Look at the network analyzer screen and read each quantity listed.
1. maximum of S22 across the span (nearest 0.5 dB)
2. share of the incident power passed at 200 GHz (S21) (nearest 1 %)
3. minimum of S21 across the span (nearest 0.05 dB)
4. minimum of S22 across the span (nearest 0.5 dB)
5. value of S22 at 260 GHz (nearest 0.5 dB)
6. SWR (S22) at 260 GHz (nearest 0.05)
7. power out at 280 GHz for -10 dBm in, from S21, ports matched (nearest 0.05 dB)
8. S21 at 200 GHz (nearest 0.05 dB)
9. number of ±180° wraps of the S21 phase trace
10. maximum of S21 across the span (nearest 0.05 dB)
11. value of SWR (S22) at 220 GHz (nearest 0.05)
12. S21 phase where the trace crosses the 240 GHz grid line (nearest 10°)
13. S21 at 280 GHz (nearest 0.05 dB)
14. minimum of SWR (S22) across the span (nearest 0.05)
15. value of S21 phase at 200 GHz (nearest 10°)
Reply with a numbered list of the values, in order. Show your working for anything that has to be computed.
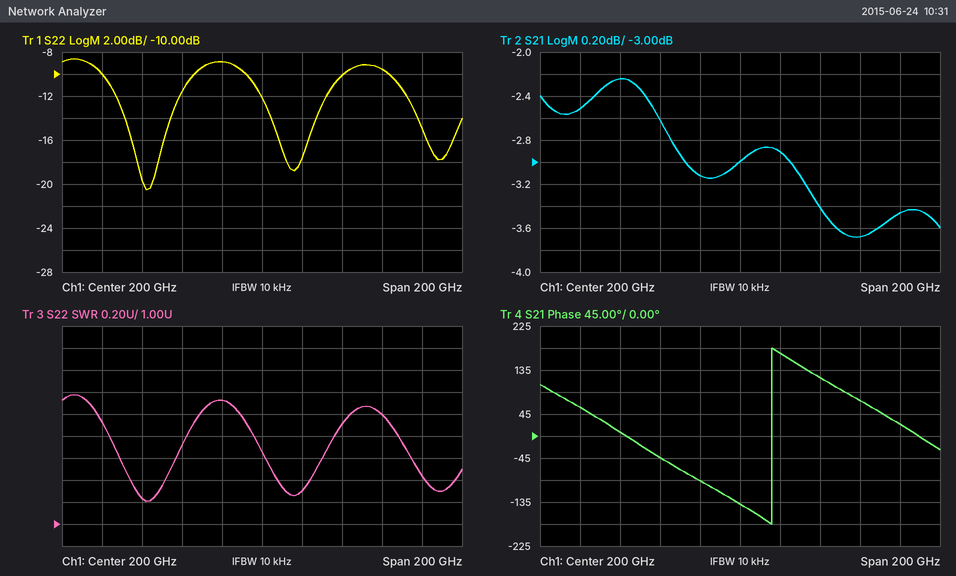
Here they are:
1. -8.5 dB
2. 10^(-3/10) ≈ 50 %
3. -3.70 dB
4. -20.5 dB
5. -9.5 dB
6. 2.00
7. -10 dBm + (-3.45 dB) = -13.45 dBm
8. -3.00 dB
9. 1
10. -2.25 dB
11. 1.30
12. 120°
13. -3.45 dB
14. 1.20
15. -140°
